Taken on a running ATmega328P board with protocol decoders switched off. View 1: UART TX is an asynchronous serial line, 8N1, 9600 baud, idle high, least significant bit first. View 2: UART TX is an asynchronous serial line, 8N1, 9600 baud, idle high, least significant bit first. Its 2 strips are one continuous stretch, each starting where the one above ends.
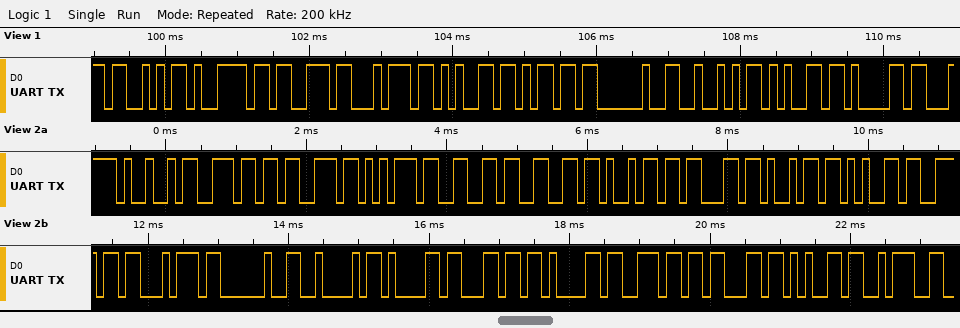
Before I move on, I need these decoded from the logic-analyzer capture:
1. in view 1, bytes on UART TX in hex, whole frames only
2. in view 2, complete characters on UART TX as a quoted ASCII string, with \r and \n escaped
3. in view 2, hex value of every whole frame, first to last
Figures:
0x53 0x79 0x73 0x74 0x65 0x6D 0x20 0x52 0x65 0x61
"Insufficient Balance:"
49 6E 73 75 66 66 69 63 69 65 6E 74 20 42 61 6C 61 6E 63 65 3A
